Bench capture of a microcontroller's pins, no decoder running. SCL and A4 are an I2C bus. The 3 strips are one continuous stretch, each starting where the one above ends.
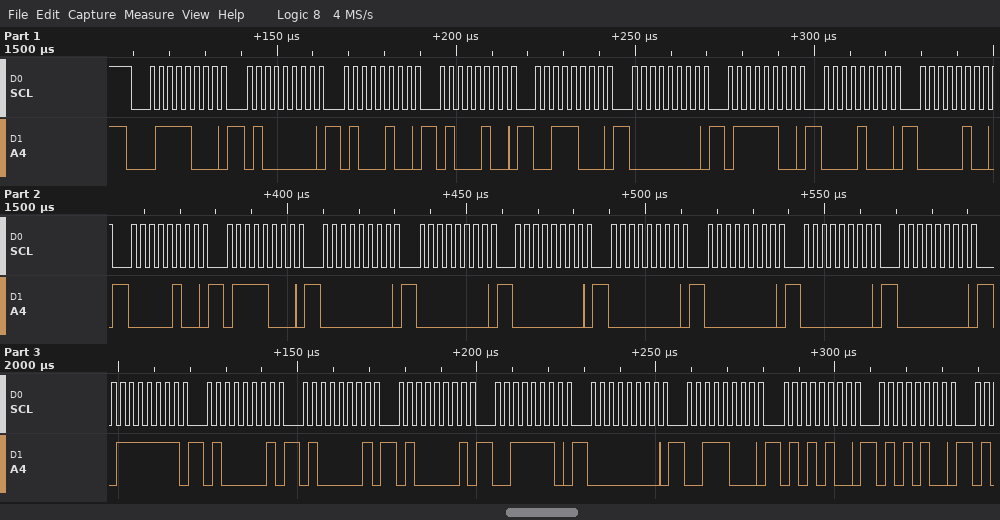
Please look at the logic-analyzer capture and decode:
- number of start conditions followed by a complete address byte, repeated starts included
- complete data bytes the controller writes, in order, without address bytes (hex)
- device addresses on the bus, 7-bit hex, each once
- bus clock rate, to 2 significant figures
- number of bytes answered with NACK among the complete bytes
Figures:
1
40 44 44 38 00 7C 08 04 04 78 00 00 00 00 00 00 00 7F 41 41 41 3E 00 38 54 54
0x3C
400 kHz
0
